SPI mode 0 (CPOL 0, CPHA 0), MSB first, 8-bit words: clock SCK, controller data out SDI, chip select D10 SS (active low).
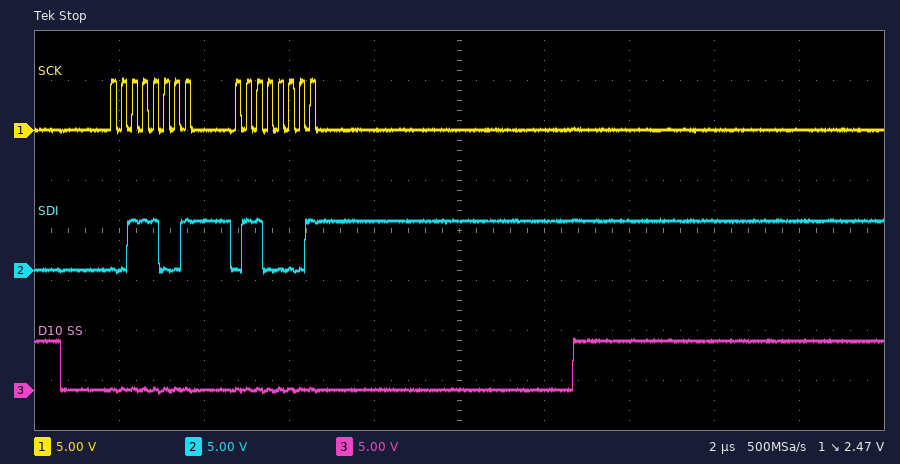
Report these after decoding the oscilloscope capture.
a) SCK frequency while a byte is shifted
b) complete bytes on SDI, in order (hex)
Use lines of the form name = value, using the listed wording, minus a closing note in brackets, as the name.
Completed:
SCK frequency while a byte is shifted = 4 MHz
complete bytes on SDI, in order = 39 61
